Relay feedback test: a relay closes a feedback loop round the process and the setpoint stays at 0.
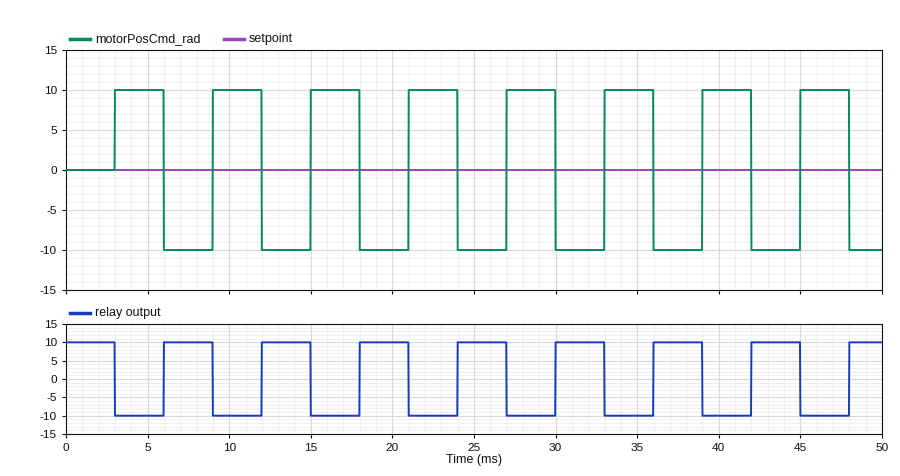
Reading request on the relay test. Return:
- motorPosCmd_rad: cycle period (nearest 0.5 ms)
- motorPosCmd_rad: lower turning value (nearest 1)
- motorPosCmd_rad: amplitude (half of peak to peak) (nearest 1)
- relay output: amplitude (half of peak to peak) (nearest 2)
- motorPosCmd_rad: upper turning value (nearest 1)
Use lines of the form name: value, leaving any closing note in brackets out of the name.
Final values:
motorPosCmd_rad: cycle period: 6.0 ms
motorPosCmd_rad: lower turning value: -10
motorPosCmd_rad: amplitude (half of peak to peak): 10
relay output: amplitude (half of peak to peak): 10
motorPosCmd_rad: upper turning value: 10
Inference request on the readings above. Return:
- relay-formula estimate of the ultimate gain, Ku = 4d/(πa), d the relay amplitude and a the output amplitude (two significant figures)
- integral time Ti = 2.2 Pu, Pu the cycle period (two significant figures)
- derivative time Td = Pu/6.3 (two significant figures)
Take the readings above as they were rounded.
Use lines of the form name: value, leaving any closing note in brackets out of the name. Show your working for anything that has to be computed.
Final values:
relay-formula estimate of the ultimate gain, Ku = 4d/(πa), d the relay amplitude and a the output amplitude: 4 × 10 / (π × 10) = 1.3
integral time Ti = 2.2 Pu, Pu the cycle period: 2.2 × 6 = 13 ms
derivative time Td = Pu/6.3: 6 / 6.3 = 0.95 ms
